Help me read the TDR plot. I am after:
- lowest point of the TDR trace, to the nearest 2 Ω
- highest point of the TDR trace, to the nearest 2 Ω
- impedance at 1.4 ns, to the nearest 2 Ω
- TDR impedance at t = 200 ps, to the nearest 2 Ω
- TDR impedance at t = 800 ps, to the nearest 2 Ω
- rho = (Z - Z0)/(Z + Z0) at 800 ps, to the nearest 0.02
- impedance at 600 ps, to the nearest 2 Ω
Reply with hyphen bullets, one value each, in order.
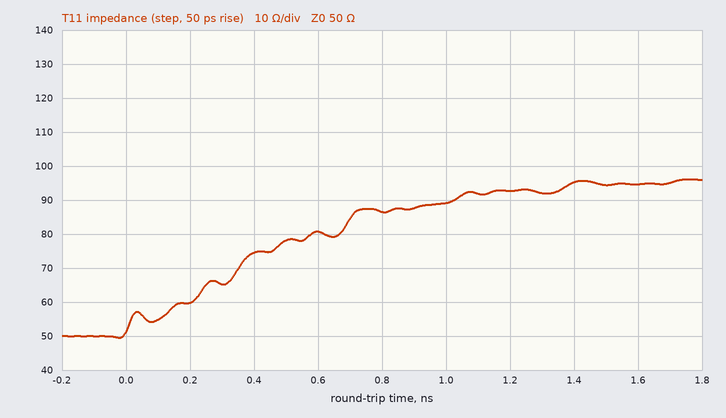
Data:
- 50 Ω
- 96 Ω
- 96 Ω
- 60 Ω
- 86 Ω
- +0.26
- 80 Ω
